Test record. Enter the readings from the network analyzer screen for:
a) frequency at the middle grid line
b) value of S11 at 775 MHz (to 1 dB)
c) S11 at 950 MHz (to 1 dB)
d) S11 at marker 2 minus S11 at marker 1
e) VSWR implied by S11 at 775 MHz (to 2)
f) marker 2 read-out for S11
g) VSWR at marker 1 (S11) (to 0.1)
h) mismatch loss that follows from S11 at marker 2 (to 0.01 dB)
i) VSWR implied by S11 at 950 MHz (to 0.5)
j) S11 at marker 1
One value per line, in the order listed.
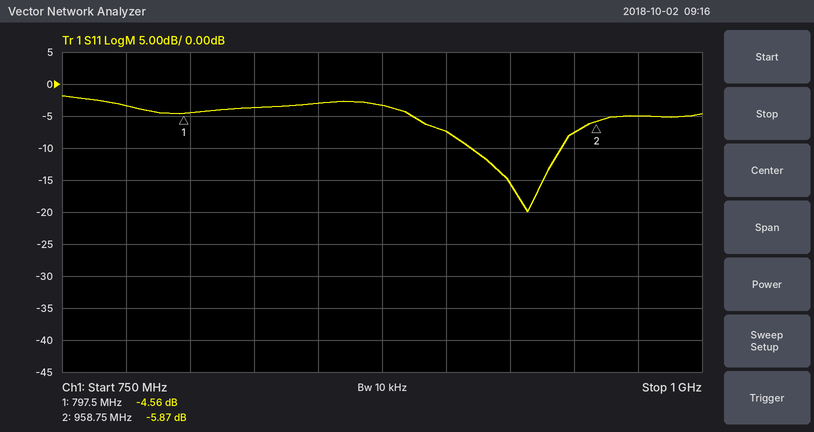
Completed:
875 MHz
-3 dB
-8 dB
-1.31 dB
6
-5.87 dB
3.9
1.30 dB
2.5
-4.56 dB
